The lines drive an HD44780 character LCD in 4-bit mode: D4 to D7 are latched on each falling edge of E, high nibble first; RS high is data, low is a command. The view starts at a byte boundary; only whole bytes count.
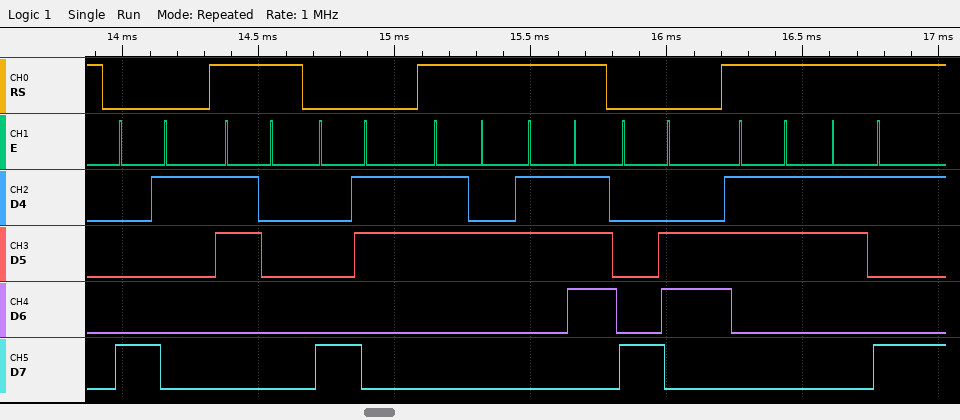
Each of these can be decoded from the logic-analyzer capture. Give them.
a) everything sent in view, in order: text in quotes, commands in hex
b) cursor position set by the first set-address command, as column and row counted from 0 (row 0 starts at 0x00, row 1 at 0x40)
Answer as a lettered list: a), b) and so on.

a) 0x81 "0" 0x83 "27" 0x86 "39"
b) column 1, row 0
